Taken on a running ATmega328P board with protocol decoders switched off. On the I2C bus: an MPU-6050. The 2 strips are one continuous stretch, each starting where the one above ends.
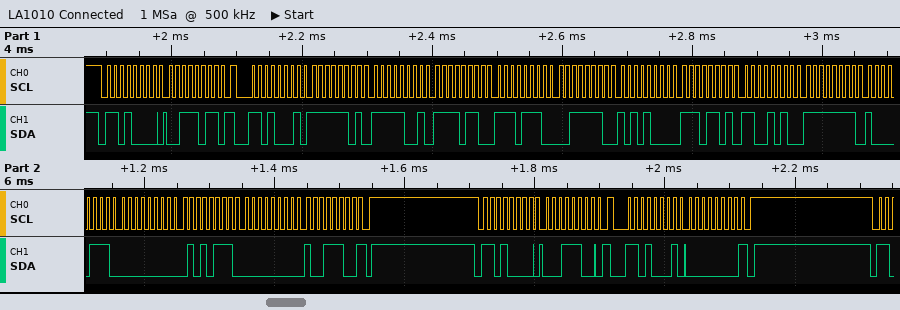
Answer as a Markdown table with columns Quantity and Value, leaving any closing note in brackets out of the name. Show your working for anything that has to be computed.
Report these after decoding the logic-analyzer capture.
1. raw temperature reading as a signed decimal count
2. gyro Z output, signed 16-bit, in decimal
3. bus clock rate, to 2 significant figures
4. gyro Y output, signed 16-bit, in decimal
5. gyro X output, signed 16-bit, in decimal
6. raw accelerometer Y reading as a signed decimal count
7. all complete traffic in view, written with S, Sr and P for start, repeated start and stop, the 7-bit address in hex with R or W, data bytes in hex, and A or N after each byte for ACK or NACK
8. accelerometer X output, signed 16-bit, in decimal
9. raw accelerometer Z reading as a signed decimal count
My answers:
| Quantity | Value |
|---|---|
| raw temperature reading as a signed decimal count | 0xEDCA = -4662 |
| gyro Z output, signed 16-bit, in decimal | 0x009C = 156 |
| bus clock rate, to 2 significant figures | 100 kHz |
| gyro Y output, signed 16-bit, in decimal | 0x0057 = 87 |
| gyro X output, signed 16-bit, in decimal | 0xFF87 = -121 |
| raw accelerometer Y reading as a signed decimal count | 0xF6EE = -2322 |
| all complete traffic in view, written with S, Sr and P for start, repeated start and stop, the 7-bit address in hex with R or W, data bytes in hex, and A or N after each byte for ACK or NACK | S 68W A 3B A Sr 68R A FD A F9 A F6 A EE A 3E A A8 A ED A CA A FF A 87 A 00 A 57 A 00 A 9C N P S 68W A 1C A Sr 68R A 00 N P |
| accelerometer X output, signed 16-bit, in decimal | 0xFDF9 = -519 |
| raw accelerometer Z reading as a signed decimal count | 0x3EA8 = 16040 |
